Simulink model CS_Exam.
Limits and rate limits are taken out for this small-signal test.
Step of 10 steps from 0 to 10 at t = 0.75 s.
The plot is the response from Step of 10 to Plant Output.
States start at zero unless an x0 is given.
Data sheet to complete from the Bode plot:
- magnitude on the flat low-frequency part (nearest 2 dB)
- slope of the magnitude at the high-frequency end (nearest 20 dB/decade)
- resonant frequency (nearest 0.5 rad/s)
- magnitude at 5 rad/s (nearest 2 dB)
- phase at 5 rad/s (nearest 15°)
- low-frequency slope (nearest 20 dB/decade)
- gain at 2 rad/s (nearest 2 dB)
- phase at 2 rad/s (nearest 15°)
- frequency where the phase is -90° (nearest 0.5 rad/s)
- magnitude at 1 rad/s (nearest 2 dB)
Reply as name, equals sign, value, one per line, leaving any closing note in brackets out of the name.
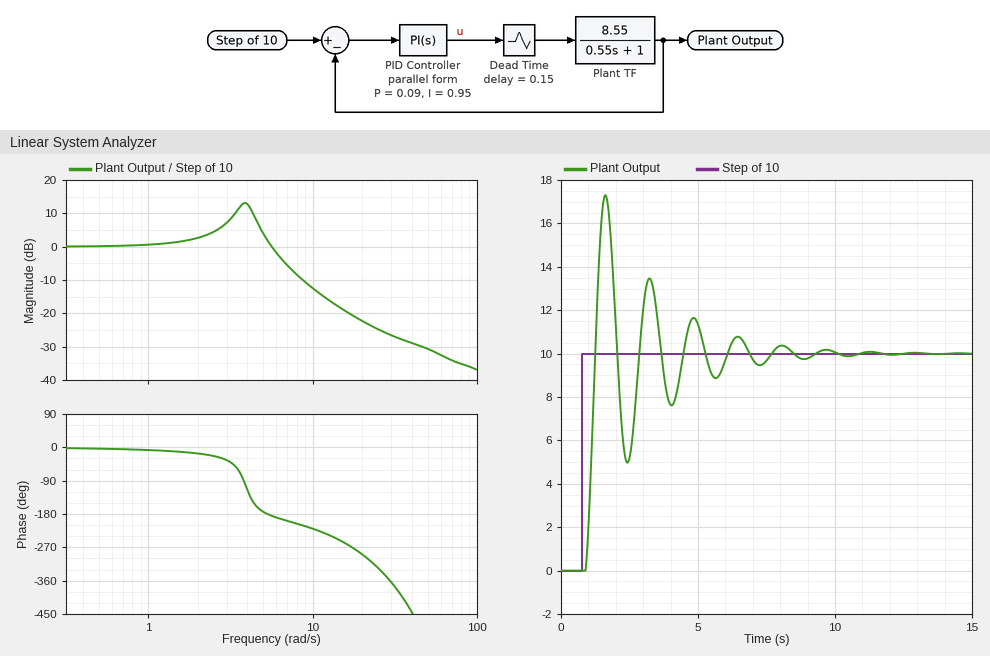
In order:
magnitude on the flat low-frequency part = 0 dB
slope of the magnitude at the high-frequency end = -20 dB/decade
resonant frequency = 4.0 rad/s
magnitude at 5 rad/s = 4 dB
phase at 5 rad/s = -180°
low-frequency slope = 0 dB/decade
gain at 2 rad/s = 2 dB
phase at 2 rad/s = -15°
frequency where the phase is -90° = 4.0 rad/s
magnitude at 1 rad/s = 0 dB
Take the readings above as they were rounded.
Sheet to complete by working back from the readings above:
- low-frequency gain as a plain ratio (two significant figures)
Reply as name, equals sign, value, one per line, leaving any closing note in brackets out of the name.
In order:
low-frequency gain as a plain ratio = 1.0
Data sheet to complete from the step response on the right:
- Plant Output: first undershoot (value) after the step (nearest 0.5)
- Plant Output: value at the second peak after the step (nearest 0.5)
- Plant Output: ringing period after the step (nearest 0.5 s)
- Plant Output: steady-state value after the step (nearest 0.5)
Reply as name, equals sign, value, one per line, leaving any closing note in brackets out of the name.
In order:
Plant Output: first undershoot (value) after the step = 5.0
Plant Output: value at the second peak after the step = 13.5
Plant Output: ringing period after the step = 1.5 s
Plant Output: steady-state value after the step = 10.0
